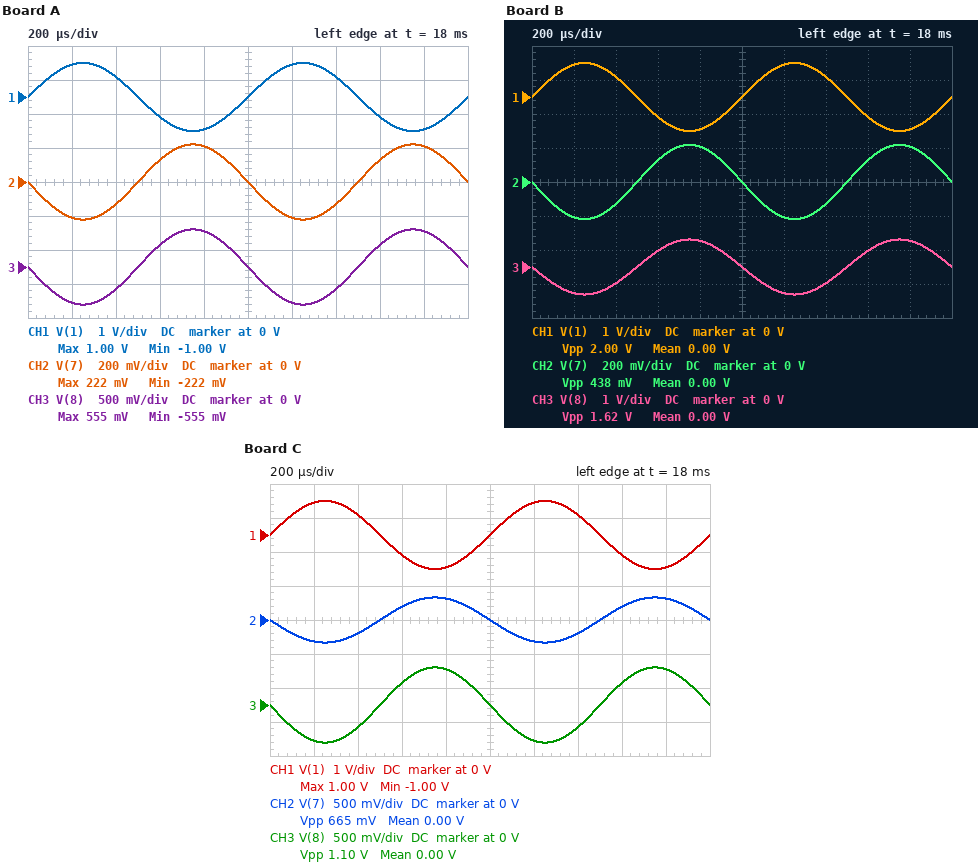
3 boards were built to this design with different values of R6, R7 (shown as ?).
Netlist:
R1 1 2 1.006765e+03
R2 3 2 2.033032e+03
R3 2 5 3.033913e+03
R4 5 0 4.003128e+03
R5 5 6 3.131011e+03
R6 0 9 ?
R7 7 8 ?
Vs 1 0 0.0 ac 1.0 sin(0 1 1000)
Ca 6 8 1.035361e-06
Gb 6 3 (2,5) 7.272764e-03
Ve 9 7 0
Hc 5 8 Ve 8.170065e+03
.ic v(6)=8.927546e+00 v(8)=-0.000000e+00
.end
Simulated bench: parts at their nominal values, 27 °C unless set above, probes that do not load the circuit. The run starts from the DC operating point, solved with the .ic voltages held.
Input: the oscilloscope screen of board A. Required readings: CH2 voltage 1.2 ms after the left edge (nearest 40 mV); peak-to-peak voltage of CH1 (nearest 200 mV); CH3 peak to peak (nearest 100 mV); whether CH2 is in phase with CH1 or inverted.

-200 mV
2.0 V
1.1 V
inverted
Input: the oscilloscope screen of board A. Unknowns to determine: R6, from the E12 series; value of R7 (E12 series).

1.2 kΩ
1.8 kΩ
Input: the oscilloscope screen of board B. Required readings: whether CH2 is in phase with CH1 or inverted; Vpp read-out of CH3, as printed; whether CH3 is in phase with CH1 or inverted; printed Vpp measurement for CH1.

inverted
1.62 V
inverted
2.00 V
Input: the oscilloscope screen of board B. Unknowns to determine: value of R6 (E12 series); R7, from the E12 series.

1 kΩ
2.7 kΩ
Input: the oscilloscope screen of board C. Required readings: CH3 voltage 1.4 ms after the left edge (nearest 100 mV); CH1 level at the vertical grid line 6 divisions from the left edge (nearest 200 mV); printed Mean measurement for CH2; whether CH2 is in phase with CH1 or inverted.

-300 mV
1.0 V
0.00 V
inverted
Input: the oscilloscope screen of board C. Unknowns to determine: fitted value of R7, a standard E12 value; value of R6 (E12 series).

1.2 kΩ
1.8 kΩ
